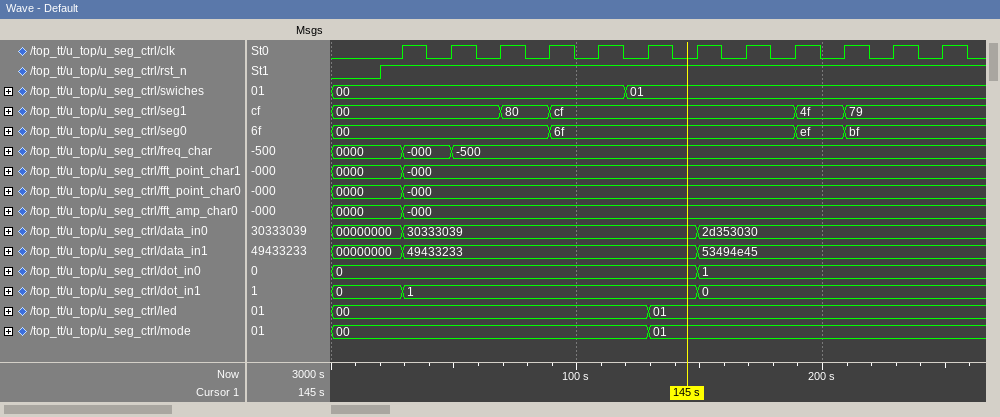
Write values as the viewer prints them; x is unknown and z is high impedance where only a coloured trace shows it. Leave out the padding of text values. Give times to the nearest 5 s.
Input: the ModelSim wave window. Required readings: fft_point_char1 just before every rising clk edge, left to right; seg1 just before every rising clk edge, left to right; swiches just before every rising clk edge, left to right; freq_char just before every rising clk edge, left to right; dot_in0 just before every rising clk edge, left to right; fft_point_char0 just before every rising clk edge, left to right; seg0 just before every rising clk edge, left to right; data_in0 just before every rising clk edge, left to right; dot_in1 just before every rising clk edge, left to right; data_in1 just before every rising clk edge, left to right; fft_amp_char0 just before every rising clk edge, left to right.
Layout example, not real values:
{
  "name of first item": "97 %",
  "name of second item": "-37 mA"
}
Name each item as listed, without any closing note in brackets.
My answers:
{
  "fft_point_char1 just before every rising clk edge, left to right": "0000, -000, -000, -000, -000, -000, -000, -000, -000, -000, -000, -000",
  "seg1 just before every rising clk edge, left to right": "00, 00, 00, 80, cf, cf, cf, cf, cf, 4f, 79, 79",
  "swiches just before every rising clk edge, left to right": "00, 00, 00, 00, 00, 01, 01, 01, 01, 01, 01, 01",
  "freq_char just before every rising clk edge, left to right": "0000, -000, -500, -500, -500, -500, -500, -500, -500, -500, -500, -500",
  "dot_in0 just before every rising clk edge, left to right": "0, 0, 0, 0, 0, 0, 0, 1, 1, 1, 1, 1",
  "fft_point_char0 just before every rising clk edge, left to right": "0000, -000, -000, -000, -000, -000, -000, -000, -000, -000, -000, -000",
  "seg0 just before every rising clk edge, left to right": "00, 00, 00, 00, 6f, 6f, 6f, 6f, 6f, ef, bf, bf",
  "data_in0 just before every rising clk edge, left to right": "00000000, 30333039, 30333039, 30333039, 30333039, 30333039, 30333039, 2d353030, 2d353030, 2d353030, 2d353030, 2d353030",
  "dot_in1 just before every rising clk edge, left to right": "0, 1, 1, 1, 1, 1, 1, 0, 0, 0, 0, 0",
  "data_in1 just before every rising clk edge, left to right": "00000000, 49433233, 49433233, 49433233, 49433233, 49433233, 49433233, 53494e45, 53494e45, 53494e45, 53494e45, 53494e45",
  "fft_amp_char0 just before every rising clk edge, left to right": "0000, -000, -000, -000, -000, -000, -000, -000, -000, -000, -000, -000"
}
